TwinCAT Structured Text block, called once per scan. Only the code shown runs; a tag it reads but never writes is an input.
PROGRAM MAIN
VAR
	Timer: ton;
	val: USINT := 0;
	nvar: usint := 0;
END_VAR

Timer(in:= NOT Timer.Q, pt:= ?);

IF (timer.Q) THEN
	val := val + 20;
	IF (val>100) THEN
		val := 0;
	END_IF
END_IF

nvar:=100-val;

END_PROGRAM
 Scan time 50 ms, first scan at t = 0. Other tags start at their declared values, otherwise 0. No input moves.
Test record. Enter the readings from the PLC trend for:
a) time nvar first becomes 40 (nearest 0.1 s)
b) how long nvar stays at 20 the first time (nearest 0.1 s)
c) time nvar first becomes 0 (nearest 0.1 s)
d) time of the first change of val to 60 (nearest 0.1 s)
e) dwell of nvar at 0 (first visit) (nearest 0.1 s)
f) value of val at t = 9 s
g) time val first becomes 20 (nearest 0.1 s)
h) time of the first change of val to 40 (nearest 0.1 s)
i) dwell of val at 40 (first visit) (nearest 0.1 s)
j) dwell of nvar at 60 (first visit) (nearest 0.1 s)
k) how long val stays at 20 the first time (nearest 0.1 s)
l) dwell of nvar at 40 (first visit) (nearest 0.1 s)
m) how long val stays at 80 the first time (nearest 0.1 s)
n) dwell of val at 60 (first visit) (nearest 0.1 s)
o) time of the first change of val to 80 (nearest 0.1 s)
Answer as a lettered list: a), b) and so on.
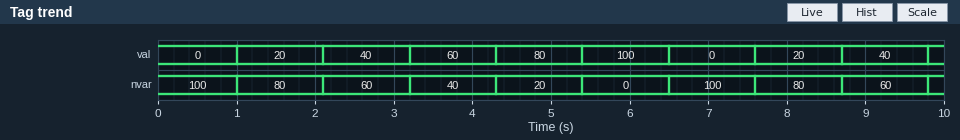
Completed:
a) 3.2 s
b) 1.1 s
c) 5.4 s
d) 3.2 s
e) 1.1 s
f) 40
g) 1.0 s
h) 2.1 s
i) 1.1 s
j) 1.1 s
k) 1.1 s
l) 1.1 s
m) 1.1 s
n) 1.1 s
o) 4.3 s
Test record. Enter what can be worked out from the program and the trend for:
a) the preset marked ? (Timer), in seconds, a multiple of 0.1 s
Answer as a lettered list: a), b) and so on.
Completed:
a) 1.0 s
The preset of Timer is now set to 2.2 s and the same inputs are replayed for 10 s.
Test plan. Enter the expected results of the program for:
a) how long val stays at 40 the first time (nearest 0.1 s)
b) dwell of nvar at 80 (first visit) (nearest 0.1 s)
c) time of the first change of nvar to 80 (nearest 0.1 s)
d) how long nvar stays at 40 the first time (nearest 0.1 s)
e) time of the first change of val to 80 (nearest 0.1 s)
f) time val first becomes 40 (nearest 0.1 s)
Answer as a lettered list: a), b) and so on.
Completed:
a) 2.3 s
b) 2.3 s
c) 2.2 s
d) 2.3 s
e) 9.1 s
f) 4.5 s
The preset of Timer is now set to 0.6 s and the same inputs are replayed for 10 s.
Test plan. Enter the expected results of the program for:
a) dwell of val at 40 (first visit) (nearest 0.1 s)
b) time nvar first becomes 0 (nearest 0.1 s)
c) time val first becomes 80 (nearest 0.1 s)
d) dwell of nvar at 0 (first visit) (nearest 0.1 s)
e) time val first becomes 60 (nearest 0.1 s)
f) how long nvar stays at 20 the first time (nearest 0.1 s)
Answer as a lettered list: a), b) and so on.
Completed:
a) 0.7 s
b) 3.4 s
c) 2.7 s
d) 0.7 s
e) 2.0 s
f) 0.7 s
